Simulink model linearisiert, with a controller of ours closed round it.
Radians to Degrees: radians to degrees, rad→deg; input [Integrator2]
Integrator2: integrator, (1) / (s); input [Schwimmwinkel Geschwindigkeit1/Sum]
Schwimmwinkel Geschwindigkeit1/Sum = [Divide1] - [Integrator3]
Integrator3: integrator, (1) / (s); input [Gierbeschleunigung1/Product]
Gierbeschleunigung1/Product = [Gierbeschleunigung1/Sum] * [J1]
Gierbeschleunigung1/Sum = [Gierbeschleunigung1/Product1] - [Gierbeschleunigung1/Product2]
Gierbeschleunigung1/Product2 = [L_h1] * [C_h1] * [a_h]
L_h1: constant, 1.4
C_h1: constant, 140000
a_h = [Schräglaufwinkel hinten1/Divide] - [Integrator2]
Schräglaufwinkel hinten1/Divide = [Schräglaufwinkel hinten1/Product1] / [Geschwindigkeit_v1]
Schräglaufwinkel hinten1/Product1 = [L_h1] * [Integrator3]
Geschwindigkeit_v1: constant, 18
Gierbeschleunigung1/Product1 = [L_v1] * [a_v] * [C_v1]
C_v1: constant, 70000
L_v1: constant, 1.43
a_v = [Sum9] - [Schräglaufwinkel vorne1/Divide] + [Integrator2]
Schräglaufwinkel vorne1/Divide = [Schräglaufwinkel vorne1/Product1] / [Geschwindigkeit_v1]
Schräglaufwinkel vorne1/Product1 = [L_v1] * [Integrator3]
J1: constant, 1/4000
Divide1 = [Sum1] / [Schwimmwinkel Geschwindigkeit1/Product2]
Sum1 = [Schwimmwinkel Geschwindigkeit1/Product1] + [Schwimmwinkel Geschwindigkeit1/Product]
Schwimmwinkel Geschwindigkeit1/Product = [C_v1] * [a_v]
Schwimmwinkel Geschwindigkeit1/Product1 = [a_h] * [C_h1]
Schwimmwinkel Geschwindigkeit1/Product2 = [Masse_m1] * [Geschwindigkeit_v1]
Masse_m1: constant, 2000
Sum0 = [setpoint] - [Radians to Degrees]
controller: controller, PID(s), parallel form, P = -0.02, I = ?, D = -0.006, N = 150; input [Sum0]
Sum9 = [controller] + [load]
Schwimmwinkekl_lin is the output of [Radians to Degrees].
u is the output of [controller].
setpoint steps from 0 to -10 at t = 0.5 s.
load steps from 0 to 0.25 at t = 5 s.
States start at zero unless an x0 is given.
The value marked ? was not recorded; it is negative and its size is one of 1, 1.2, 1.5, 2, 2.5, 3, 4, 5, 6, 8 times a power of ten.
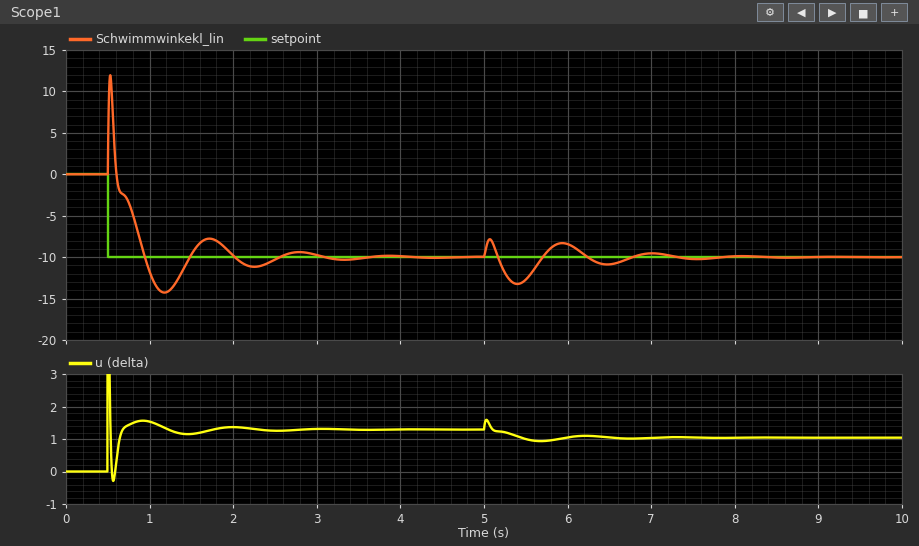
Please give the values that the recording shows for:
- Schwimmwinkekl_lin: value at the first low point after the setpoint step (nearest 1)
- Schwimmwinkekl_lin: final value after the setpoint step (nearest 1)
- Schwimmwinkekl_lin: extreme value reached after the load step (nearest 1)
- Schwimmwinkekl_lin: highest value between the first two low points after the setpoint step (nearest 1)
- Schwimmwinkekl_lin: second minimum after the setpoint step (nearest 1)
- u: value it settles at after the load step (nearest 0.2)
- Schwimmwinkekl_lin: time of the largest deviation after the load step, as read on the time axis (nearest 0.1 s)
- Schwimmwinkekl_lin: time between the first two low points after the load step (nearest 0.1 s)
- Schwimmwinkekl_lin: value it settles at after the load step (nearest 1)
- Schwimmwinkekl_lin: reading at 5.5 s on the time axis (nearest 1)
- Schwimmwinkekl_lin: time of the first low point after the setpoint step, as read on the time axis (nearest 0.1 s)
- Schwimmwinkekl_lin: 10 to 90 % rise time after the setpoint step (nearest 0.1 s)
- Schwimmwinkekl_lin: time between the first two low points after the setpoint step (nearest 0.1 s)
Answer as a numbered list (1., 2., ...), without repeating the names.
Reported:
1. -14
2. -10
3. -13
4. -8
5. -11
6. 1.0
7. 5.4 s
8. 1.1 s
9. -10
10. -13
11. 1.2 s
12. 0.3 s
13. 1.1 s
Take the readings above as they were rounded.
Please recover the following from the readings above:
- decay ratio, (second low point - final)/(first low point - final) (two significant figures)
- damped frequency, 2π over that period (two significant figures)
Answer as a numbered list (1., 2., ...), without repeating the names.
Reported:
1. 0.25
2. 5.7 rad/s
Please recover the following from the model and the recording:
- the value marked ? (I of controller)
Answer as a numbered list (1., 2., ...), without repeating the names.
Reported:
1. -0.5
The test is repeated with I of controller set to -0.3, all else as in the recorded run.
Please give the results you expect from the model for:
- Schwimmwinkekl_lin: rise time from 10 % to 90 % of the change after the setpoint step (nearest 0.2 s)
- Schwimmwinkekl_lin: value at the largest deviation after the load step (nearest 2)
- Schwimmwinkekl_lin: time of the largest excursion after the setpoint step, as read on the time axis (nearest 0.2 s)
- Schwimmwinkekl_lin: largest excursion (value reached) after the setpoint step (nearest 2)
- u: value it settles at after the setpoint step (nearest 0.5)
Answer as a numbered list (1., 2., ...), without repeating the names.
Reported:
1. 0.6 s
2. -12
3. 1.6 s
4. -10
5. 1.5
